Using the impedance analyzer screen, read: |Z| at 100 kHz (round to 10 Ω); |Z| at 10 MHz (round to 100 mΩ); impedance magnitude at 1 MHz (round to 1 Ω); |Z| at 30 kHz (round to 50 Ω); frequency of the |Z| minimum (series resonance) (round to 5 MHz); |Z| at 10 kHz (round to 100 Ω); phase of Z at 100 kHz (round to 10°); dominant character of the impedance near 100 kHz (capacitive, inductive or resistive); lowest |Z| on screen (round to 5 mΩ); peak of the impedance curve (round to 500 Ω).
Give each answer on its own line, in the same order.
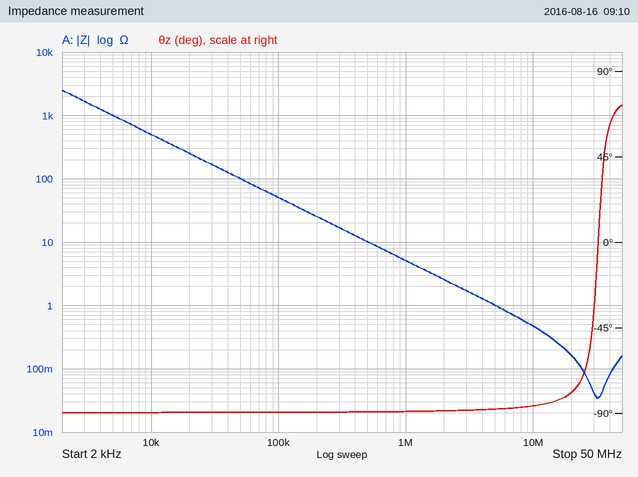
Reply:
50 Ω
500 mΩ
5 Ω
150 Ω
30 MHz
500 Ω
-90°
capacitive
35 mΩ
2.5 kΩ
